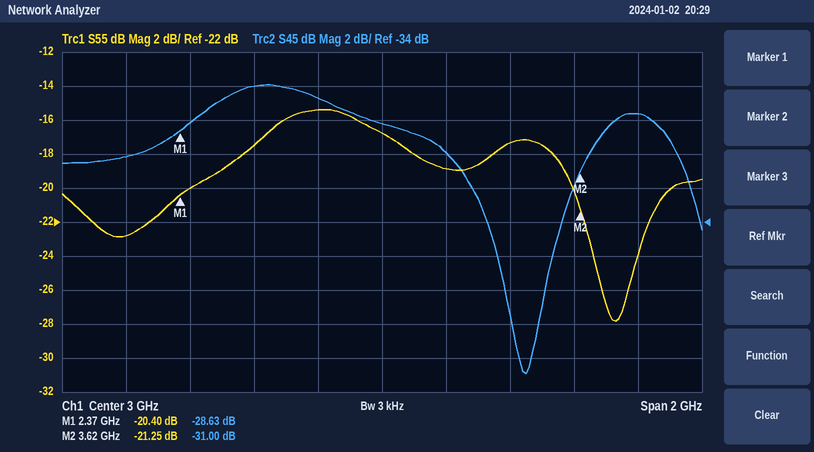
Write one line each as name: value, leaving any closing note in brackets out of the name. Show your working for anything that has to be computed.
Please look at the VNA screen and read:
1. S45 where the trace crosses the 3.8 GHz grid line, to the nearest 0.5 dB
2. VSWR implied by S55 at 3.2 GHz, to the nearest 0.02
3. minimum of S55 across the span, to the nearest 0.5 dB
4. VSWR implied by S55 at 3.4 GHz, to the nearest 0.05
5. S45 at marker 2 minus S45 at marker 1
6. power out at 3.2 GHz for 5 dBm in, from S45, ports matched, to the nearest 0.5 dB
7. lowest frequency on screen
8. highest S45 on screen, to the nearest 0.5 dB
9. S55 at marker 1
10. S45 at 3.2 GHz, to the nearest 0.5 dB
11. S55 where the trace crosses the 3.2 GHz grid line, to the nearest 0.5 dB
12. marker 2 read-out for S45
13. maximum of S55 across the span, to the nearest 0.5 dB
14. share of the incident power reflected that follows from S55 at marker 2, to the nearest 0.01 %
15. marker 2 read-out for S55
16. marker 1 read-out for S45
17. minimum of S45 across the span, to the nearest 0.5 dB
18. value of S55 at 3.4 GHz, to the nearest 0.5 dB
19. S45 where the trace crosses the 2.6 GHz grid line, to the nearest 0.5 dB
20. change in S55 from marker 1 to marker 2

S45 where the trace crosses the 3.8 GHz grid line, to the nearest 0.5 dB: -27.5 dB
VSWR implied by S55 at 3.2 GHz, to the nearest 0.02: |Γ| = 10^(-19/20) = 0.1122; VSWR = (1 + 0.1122)/(1 − 0.1122) ≈ 1.25, so 1.26 to the nearest 0.02
minimum of S55 across the span, to the nearest 0.5 dB: -28.0 dB
VSWR implied by S55 at 3.4 GHz, to the nearest 0.05: |Γ| = 10^(-17.5/20) = 0.1334; VSWR = (1 + 0.1334)/(1 − 0.1334) ≈ 1.31, so 1.30 to the nearest 0.05
S45 at marker 2 minus S45 at marker 1: -31 − (-28.63) = -2.37 dB
power out at 3.2 GHz for 5 dBm in, from S45, ports matched, to the nearest 0.5 dB: 5 dBm + (-30.0 dB) = -25.0 dBm
lowest frequency on screen: 2 GHz
highest S45 on screen, to the nearest 0.5 dB: -26.0 dB
S55 at marker 1: -20.40 dB
S45 at 3.2 GHz, to the nearest 0.5 dB: -30.0 dB
S55 where the trace crosses the 3.2 GHz grid line, to the nearest 0.5 dB: -19.0 dB
marker 2 read-out for S45: -31.00 dB
maximum of S55 across the span, to the nearest 0.5 dB: -15.5 dB
share of the incident power reflected that follows from S55 at marker 2, to the nearest 0.01 %: 10^(-21.25/10) ≈ 0.75 %
marker 2 read-out for S55: -21.25 dB
marker 1 read-out for S45: -28.63 dB
minimum of S45 across the span, to the nearest 0.5 dB: -43.0 dB
value of S55 at 3.4 GHz, to the nearest 0.5 dB: -17.5 dB
S45 where the trace crosses the 2.6 GHz grid line, to the nearest 0.5 dB: -26.0 dB
change in S55 from marker 1 to marker 2: -21.25 − (-20.4) = -0.85 dB
